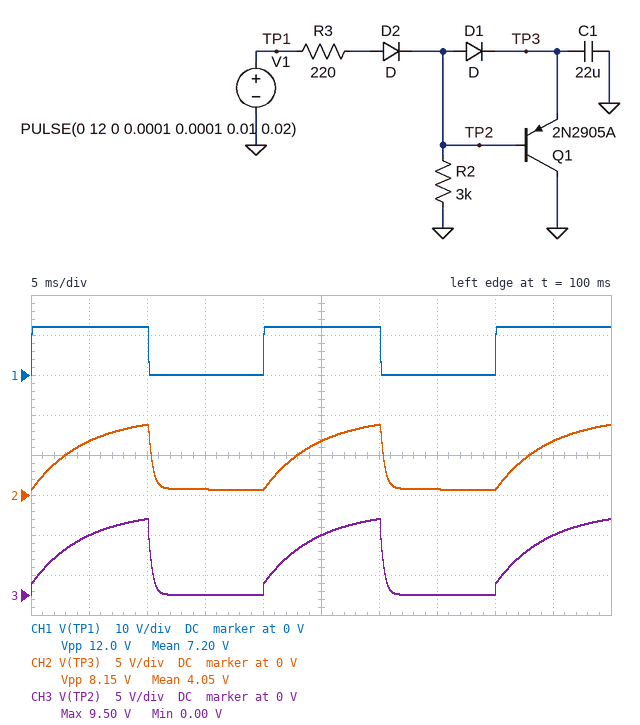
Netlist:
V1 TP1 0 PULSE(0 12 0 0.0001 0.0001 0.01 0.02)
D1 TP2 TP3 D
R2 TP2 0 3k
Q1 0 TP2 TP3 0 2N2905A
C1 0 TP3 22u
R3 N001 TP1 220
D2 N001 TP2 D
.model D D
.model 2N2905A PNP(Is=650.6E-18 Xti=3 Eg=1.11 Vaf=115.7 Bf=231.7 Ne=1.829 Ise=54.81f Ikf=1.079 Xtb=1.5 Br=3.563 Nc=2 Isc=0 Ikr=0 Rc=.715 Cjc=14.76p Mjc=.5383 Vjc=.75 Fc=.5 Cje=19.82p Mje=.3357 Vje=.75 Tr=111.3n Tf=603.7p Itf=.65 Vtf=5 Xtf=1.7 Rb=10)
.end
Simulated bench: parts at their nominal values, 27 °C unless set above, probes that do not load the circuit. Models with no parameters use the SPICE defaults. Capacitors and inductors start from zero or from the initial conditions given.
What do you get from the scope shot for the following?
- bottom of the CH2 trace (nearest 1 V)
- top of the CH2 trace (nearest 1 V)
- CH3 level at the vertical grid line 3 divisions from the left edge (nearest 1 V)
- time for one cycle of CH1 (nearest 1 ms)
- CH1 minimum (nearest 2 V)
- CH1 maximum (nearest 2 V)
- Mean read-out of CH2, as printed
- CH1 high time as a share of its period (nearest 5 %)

1 V
9 V
0 V
20 ms
0 V
12 V
4.05 V
50 %
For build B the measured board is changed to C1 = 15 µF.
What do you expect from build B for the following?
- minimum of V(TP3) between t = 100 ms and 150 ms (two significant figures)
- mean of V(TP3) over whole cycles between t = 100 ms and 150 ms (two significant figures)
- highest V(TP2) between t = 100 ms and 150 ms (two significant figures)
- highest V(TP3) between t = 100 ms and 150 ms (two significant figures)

650 mV
4.0 V
10 V
9.5 V
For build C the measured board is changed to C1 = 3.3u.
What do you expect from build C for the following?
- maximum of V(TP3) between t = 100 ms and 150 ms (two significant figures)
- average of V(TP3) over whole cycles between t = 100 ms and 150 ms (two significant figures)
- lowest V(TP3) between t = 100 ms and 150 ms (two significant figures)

10 V
5.0 V
600 mV
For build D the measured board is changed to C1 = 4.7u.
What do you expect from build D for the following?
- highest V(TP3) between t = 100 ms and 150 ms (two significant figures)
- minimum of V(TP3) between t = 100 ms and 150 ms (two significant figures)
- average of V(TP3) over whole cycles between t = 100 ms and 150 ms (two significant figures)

10 V
610 mV
4.9 V
